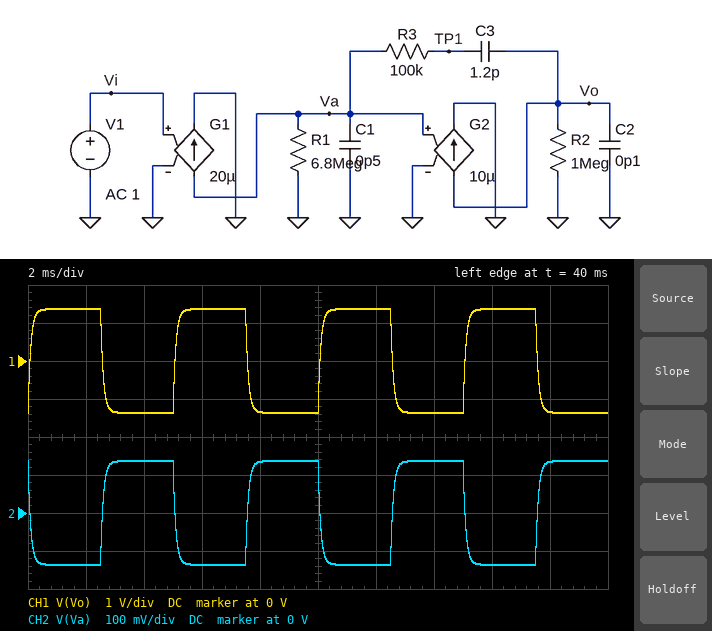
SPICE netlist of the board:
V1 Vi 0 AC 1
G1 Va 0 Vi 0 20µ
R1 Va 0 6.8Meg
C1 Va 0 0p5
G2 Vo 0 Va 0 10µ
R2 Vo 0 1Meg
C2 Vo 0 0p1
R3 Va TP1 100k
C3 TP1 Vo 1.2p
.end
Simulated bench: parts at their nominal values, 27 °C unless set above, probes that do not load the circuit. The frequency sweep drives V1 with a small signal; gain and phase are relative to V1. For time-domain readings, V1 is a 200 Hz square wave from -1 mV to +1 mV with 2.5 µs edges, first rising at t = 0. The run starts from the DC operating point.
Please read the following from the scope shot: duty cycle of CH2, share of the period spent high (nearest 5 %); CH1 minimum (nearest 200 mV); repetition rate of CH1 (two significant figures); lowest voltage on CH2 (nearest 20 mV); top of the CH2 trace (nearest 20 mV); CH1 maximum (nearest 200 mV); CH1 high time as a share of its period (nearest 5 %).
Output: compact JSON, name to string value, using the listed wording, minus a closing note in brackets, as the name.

{"duty cycle of CH2, share of the period spent high": "50 %", "CH1 minimum": "-1.4 V", "repetition rate of CH1": "200 Hz", "lowest voltage on CH2": "-140 mV", "top of the CH2 trace": "140 mV", "CH1 maximum": "1.4 V", "CH1 high time as a share of its period": "50 %"}
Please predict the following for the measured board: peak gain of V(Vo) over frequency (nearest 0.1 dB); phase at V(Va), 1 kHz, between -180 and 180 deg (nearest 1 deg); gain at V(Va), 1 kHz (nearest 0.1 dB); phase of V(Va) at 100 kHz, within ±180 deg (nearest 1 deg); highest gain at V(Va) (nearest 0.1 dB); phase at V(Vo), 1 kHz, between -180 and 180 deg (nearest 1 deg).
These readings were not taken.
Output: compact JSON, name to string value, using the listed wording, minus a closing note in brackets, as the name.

{"peak gain of V(Vo) over frequency": "62.7 dB", "phase at V(Va), 1 kHz, between -180 and 180 deg": "150 deg", "gain at V(Va), 1 kHz": "41.4 dB", "phase of V(Va) at 100 kHz, within ±180 deg": "131 deg", "highest gain at V(Va)": "42.7 dB", "phase at V(Vo), 1 kHz, between -180 and 180 deg": "-31 deg"}
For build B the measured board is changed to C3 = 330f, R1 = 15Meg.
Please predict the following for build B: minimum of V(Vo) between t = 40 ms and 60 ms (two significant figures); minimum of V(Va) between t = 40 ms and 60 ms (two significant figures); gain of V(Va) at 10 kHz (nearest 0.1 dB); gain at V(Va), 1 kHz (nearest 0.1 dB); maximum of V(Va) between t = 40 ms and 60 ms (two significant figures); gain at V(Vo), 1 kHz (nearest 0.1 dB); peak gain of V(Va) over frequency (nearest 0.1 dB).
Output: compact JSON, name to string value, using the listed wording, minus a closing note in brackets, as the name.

{"minimum of V(Vo) between t = 40 ms and 60 ms": "-3.0 V", "minimum of V(Va) between t = 40 ms and 60 ms": "-300 mV", "gain of V(Va) at 10 kHz": "37.4 dB", "gain at V(Va), 1 kHz": "48.9 dB", "maximum of V(Va) between t = 40 ms and 60 ms": "300 mV", "gain at V(Vo), 1 kHz": "68.9 dB", "peak gain of V(Va) over frequency": "49.5 dB"}
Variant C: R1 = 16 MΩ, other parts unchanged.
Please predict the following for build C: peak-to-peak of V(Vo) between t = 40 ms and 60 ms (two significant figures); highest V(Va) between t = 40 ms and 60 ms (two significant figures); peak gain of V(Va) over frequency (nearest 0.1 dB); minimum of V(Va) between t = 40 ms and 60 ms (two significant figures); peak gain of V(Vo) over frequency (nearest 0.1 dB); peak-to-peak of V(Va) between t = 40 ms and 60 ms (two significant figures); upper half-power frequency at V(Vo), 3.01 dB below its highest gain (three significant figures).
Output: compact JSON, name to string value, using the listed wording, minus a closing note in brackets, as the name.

{"peak-to-peak of V(Vo) between t = 40 ms and 60 ms": "6.4 V", "highest V(Va) between t = 40 ms and 60 ms": "320 mV", "peak gain of V(Va) over frequency": "50.1 dB", "minimum of V(Va) between t = 40 ms and 60 ms": "-320 mV", "peak gain of V(Vo) over frequency": "70.1 dB", "peak-to-peak of V(Va) between t = 40 ms and 60 ms": "640 mV", "upper half-power frequency at V(Vo), 3.01 dB below its highest gain": "722 Hz"}
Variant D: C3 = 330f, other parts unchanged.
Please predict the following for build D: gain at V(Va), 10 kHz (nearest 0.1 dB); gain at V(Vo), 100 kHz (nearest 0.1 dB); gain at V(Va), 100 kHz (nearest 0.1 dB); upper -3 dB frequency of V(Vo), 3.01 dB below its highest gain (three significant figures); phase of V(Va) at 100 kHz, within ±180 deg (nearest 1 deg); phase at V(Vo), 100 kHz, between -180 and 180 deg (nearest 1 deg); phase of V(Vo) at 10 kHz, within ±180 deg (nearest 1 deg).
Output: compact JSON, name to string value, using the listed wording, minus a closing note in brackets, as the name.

{"gain at V(Va), 10 kHz": "36.4 dB", "gain at V(Vo), 100 kHz": "37.6 dB", "gain at V(Va), 100 kHz": "17.9 dB", "upper -3 dB frequency of V(Vo), 3.01 dB below its highest gain": "5.59 kHz", "phase of V(Va) at 100 kHz, within ±180 deg": "107 deg", "phase at V(Vo), 100 kHz, between -180 and 180 deg": "-89 deg", "phase of V(Vo) at 10 kHz, within ±180 deg": "-61 deg"}
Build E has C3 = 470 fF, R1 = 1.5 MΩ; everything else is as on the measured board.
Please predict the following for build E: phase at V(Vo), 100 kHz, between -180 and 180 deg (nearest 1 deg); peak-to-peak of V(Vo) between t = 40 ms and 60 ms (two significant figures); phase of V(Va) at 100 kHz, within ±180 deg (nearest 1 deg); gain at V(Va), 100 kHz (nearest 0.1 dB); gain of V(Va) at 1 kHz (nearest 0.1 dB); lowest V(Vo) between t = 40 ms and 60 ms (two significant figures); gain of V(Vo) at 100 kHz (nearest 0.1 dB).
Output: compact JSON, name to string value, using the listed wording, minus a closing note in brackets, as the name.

{"phase at V(Vo), 100 kHz, between -180 and 180 deg": "-82 deg", "peak-to-peak of V(Vo) between t = 40 ms and 60 ms": "600 mV", "phase of V(Va) at 100 kHz, within ±180 deg": "119 deg", "gain at V(Va), 100 kHz": "14.9 dB", "gain of V(Va) at 1 kHz": "29.5 dB", "lowest V(Vo) between t = 40 ms and 60 ms": "-300 mV", "gain of V(Vo) at 100 kHz": "34.3 dB"}
